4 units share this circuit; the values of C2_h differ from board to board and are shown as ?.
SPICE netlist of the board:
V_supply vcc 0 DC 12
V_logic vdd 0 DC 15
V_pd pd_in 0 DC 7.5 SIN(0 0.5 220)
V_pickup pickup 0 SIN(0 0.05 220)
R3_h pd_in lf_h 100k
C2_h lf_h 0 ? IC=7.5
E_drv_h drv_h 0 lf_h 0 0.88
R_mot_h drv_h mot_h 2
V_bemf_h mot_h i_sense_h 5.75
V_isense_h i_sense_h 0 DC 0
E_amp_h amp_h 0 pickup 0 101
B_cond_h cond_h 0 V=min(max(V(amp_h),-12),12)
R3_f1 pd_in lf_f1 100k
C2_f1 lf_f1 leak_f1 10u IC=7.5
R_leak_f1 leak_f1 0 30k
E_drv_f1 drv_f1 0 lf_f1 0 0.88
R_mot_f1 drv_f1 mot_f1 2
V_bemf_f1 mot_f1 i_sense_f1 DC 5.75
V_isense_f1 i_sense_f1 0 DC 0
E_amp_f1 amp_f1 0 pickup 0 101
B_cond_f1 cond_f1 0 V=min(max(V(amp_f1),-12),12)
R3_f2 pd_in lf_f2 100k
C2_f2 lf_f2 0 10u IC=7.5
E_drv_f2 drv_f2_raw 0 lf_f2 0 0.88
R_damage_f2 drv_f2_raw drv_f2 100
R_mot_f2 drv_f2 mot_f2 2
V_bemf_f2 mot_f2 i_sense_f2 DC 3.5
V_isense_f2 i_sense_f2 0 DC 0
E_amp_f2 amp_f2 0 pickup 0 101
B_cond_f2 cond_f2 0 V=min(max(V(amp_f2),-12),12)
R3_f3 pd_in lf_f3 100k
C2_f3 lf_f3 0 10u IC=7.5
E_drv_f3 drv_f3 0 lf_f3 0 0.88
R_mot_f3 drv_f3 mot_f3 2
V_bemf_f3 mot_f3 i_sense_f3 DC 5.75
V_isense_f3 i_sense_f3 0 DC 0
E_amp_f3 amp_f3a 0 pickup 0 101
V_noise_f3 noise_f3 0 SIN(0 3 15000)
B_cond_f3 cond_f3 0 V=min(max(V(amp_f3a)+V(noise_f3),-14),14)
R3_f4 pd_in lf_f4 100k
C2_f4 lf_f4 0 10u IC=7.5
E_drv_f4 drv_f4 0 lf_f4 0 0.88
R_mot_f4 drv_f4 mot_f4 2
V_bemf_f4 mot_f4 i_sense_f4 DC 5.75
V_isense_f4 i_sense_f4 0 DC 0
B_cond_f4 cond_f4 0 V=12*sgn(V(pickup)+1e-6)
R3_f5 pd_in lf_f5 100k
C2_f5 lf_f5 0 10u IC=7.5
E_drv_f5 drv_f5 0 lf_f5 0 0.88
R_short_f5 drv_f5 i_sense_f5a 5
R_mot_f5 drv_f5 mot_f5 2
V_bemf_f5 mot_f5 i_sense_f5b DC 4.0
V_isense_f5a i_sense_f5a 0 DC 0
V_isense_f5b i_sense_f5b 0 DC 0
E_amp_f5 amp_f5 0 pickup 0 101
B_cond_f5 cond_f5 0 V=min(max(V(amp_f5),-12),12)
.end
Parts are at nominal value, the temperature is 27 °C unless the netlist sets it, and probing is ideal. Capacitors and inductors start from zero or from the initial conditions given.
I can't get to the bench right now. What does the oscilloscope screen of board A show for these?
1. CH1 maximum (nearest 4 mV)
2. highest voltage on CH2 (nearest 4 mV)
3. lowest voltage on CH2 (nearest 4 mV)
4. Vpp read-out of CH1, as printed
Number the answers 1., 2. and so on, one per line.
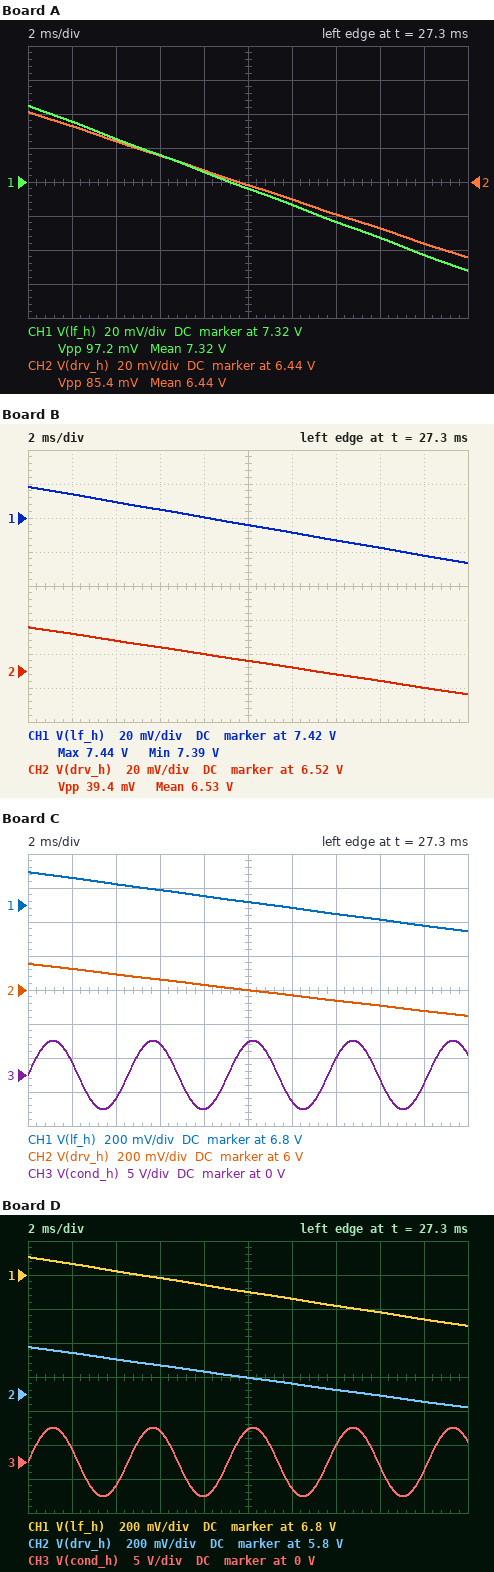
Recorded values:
1. 7.364 V
2. 6.480 V
3. 6.396 V
4. 97.2 mV
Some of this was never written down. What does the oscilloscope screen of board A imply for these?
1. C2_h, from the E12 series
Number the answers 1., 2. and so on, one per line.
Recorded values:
1. 15 µF
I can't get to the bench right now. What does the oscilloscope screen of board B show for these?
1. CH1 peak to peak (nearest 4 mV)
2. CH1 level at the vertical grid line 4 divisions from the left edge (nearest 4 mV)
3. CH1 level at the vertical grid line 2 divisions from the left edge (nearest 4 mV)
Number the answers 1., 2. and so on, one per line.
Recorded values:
1. 44 mV
2. 7.420 V
3. 7.428 V
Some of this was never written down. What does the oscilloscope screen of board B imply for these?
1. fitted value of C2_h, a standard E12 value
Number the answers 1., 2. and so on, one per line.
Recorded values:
1. 33 µF
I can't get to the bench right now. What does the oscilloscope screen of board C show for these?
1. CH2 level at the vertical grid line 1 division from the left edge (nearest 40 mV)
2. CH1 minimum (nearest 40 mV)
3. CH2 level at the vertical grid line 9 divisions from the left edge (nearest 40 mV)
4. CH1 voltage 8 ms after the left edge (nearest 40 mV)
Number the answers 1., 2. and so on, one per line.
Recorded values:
1. 6.12 V
2. 6.64 V
3. 5.88 V
4. 6.84 V
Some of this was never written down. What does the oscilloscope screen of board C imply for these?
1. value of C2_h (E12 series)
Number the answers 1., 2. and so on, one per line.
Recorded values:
1. 3.9 µF
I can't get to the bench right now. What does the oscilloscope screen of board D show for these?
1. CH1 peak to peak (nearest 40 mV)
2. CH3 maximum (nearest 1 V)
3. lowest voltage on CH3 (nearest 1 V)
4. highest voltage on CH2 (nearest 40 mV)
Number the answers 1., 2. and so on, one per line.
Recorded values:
1. 400 mV
2. 5 V
3. -5 V
4. 6.08 V
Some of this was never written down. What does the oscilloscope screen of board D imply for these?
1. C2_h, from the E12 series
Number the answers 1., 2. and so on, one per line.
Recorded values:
1. 3.3 µF
